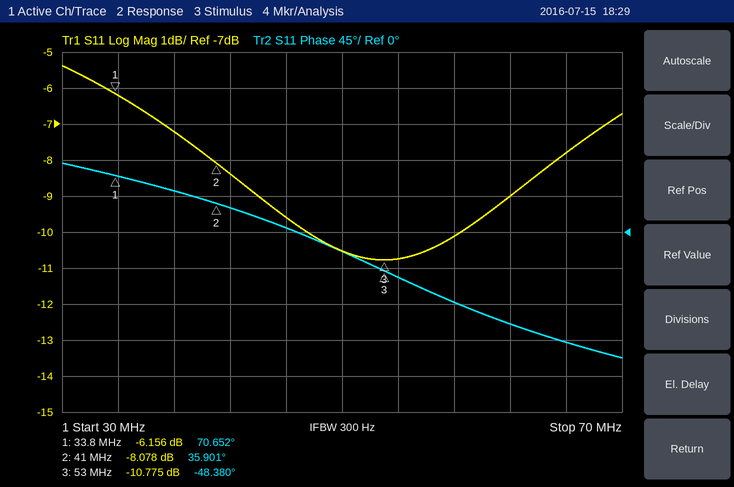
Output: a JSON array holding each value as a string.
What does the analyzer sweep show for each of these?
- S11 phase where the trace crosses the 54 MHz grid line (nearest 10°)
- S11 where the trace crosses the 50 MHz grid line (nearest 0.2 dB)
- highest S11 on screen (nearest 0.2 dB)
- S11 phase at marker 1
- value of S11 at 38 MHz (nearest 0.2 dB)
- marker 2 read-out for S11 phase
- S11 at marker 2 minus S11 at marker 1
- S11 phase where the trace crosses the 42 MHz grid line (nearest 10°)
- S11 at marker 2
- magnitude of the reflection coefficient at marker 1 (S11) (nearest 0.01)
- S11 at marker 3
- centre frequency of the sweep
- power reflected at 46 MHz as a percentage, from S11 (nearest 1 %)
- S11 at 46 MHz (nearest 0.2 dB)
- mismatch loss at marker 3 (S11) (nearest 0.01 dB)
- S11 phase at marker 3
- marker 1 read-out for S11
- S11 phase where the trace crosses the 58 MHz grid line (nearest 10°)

["-60°", "-10.6 dB", "-5.4 dB", "70.652°", "-7.2 dB", "35.901°", "-1.922 dB", "30°", "-8.078 dB", "0.49", "-10.775 dB", "50 MHz", "11 %", "-9.6 dB", "0.38 dB", "-48.380°", "-6.156 dB", "-90°"]
